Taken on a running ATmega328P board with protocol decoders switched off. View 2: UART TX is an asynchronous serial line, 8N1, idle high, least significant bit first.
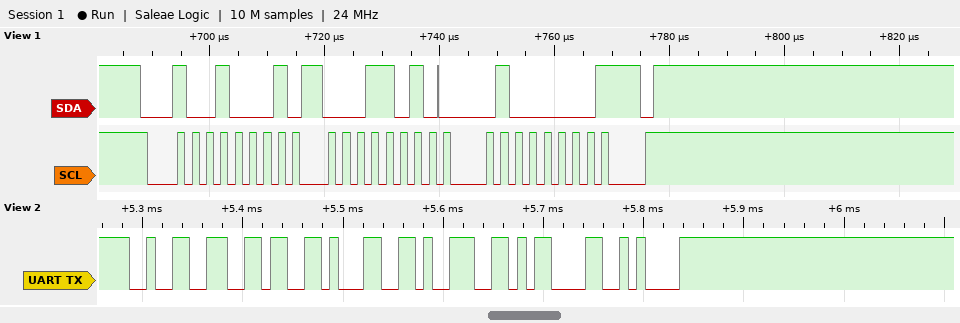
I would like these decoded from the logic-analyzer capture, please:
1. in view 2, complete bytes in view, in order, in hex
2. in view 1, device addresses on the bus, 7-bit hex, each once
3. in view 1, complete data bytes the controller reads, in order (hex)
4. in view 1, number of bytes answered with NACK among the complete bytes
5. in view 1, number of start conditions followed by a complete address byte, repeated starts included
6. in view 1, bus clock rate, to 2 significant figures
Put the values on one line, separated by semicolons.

0x32 0x36 0x31 0x39 0x0D 0x0A; 0x48; 1A 40; 1; 1; 400 kHz
